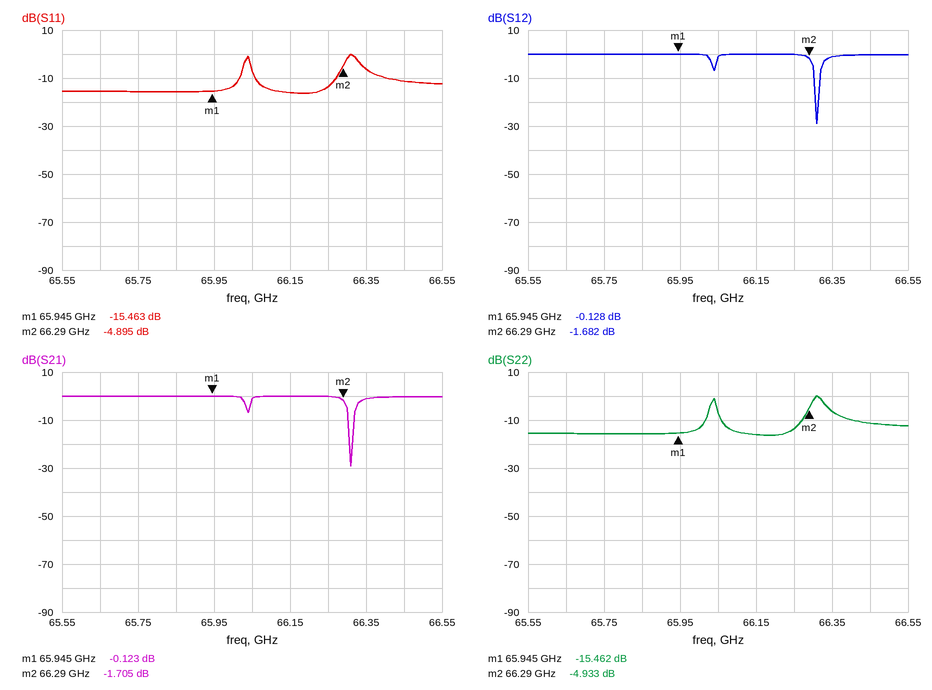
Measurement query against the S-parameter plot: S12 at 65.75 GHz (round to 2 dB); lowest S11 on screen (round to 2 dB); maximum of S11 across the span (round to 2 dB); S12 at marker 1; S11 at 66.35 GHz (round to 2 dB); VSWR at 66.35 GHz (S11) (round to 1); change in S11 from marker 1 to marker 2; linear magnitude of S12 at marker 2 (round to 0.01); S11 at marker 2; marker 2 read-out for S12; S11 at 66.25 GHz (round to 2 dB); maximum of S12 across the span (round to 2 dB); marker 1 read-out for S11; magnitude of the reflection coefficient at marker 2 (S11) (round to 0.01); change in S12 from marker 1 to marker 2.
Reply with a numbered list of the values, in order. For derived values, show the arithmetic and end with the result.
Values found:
1. 0 dB
2. -16 dB
3. 0 dB
4. -0.128 dB
5. -6 dB
6. |Γ| = 10^(-6/20) = 0.5012; VSWR = (1 + 0.5012)/(1 − 0.5012) ≈ 3
7. -4.895 − (-15.463) = 10.568 dB
8. 10^(-1.682/20) ≈ 0.82
9. -4.895 dB
10. -1.682 dB
11. -14 dB
12. 0 dB
13. -15.463 dB
14. 10^(-4.895/20) ≈ 0.57
15. -1.682 − (-0.128) = -1.554 dB
